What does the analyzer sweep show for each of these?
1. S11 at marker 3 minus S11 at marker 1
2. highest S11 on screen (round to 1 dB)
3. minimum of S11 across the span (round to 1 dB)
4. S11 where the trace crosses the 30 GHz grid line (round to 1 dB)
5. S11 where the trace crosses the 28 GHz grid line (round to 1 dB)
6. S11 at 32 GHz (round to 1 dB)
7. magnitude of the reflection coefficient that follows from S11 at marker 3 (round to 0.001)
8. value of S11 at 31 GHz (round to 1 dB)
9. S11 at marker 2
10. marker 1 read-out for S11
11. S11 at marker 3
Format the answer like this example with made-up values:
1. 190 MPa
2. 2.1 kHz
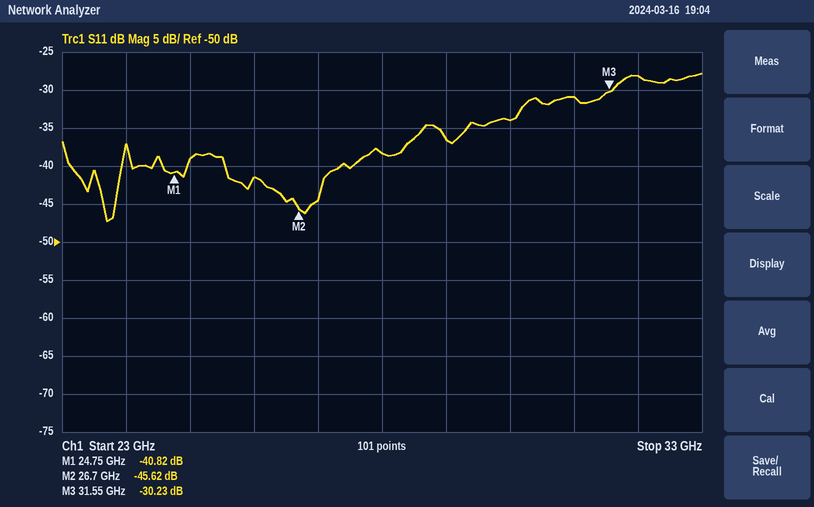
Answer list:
1. 10.59 dB
2. -28 dB
3. -47 dB
4. -34 dB
5. -38 dB
6. -28 dB
7. 0.031
8. -31 dB
9. -45.62 dB
10. -40.82 dB
11. -30.23 dB
